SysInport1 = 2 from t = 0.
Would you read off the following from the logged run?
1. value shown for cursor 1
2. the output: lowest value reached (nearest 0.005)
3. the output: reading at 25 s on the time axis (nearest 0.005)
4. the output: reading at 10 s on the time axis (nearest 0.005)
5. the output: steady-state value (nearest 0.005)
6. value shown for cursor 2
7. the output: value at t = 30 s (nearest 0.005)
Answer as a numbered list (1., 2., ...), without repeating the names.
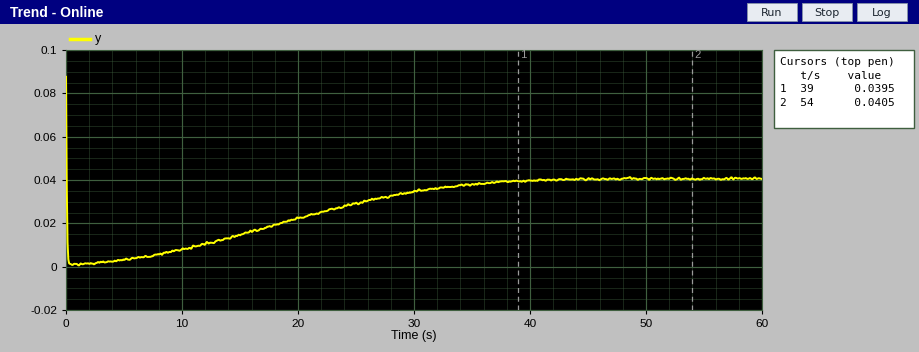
1. 0.0395
2. 0.000
3. 0.030
4. 0.010
5. 0.040
6. 0.0405
7. 0.035
